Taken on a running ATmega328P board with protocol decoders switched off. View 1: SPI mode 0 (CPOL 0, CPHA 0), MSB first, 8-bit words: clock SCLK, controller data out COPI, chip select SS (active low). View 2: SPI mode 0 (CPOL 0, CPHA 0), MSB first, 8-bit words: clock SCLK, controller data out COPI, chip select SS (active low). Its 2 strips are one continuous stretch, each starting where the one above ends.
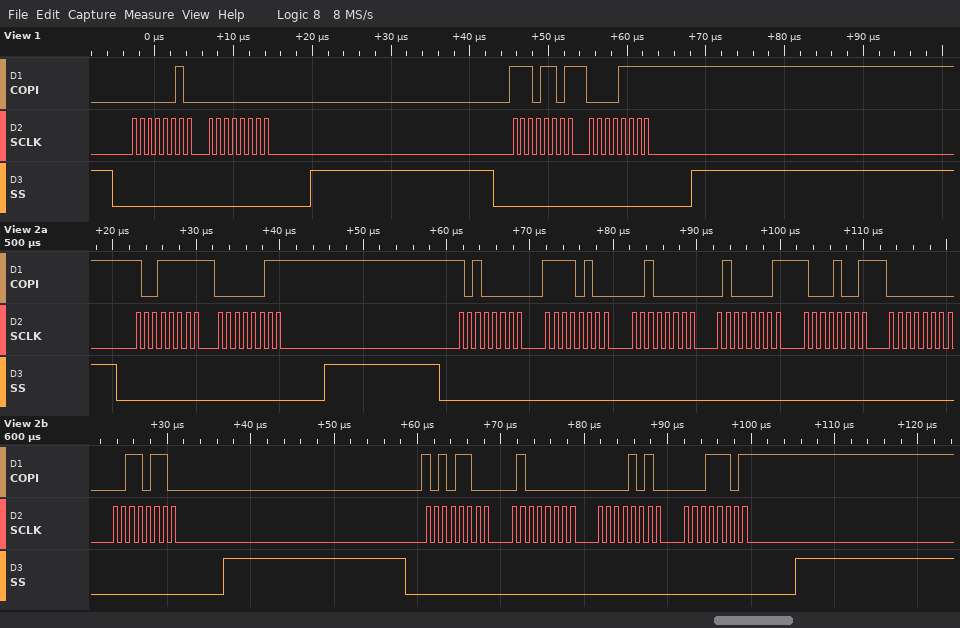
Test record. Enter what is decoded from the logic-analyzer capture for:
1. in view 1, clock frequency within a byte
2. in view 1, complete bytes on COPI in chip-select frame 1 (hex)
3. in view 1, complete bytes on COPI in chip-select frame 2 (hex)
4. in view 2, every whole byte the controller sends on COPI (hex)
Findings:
1 MHz
02 00
ED 0F
9F 03 A0 F4 20 41 89 00 36 AC 40 0A 1D
